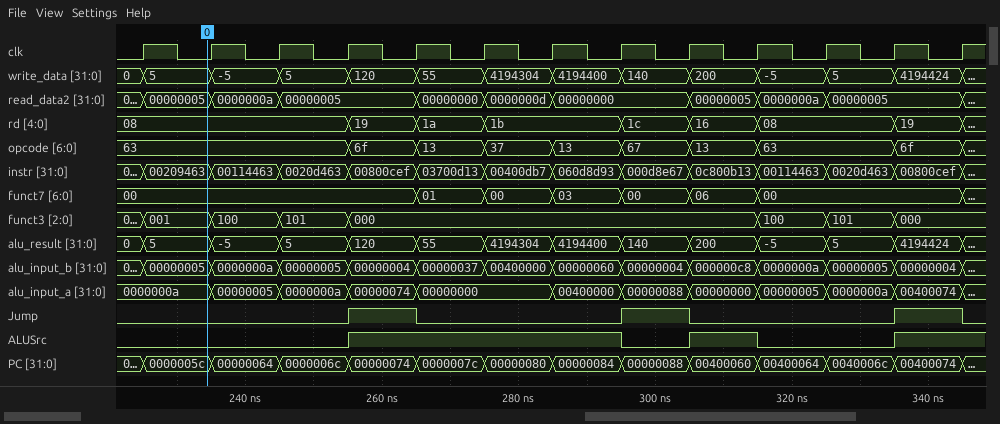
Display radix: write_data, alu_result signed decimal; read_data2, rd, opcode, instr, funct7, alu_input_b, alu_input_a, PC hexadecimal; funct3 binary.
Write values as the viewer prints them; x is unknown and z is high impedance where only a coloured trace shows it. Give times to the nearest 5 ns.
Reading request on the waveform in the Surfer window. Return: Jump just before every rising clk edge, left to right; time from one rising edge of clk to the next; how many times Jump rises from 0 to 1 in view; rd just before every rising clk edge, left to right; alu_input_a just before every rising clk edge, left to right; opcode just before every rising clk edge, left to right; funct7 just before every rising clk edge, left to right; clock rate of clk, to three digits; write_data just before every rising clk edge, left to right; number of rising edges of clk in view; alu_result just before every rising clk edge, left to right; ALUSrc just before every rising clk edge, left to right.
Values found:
0 0 0 0 1 0 0 0 1 0 0 0 1
10 ns
3
08, 08, 08, 08, 19, 1a, 1b, 1b, 1c, 16, 08, 08, 19
0000000a, 0000000a, 00000005, 0000000a, 00000074, 00000000, 00000000, 00400000, 00000088, 00000000, 00000005, 0000000a, 00400074
63, 63, 63, 63, 6f, 13, 37, 13, 67, 13, 63, 63, 6f
00, 00, 00, 00, 00, 01, 00, 03, 00, 06, 00, 00, 00
100 MHz
0, 5, -5, 5, 120, 55, 4194304, 4194400, 140, 200, -5, 5, 4194424
13
0, 5, -5, 5, 120, 55, 4194304, 4194400, 140, 200, -5, 5, 4194424
0 0 0 0 1 1 1 1 0 1 0 0 1
